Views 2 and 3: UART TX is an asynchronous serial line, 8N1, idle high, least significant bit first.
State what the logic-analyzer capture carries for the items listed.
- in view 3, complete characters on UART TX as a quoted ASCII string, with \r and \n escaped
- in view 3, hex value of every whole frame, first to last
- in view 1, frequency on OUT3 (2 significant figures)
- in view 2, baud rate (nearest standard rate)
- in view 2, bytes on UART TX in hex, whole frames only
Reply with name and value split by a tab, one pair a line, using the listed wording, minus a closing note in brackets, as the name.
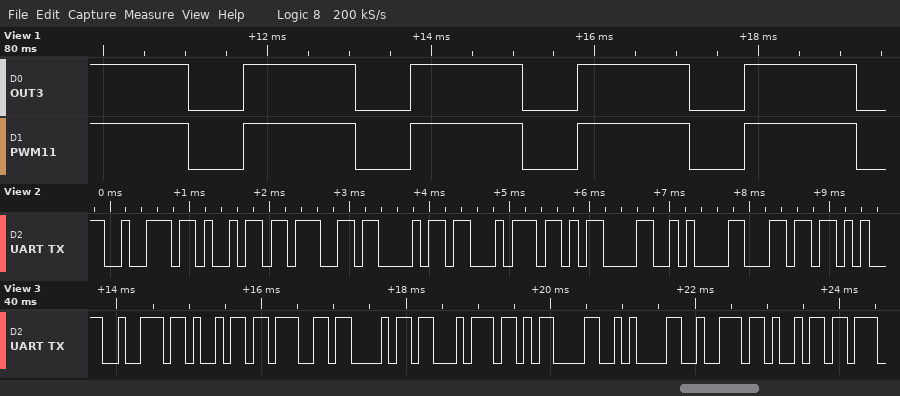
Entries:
in view 3, complete characters on UART TX as a quoted ASCII string, with \r and \n escaped	"right\r\nri"
in view 3, hex value of every whole frame, first to last	72 69 67 68 74 0D 0A 72 69
in view 1, frequency on OUT3	490 Hz
in view 2, baud rate	9600 baud
in view 2, bytes on UART TX in hex, whole frames only	72 69 67 68 74 0D 0A 6C
